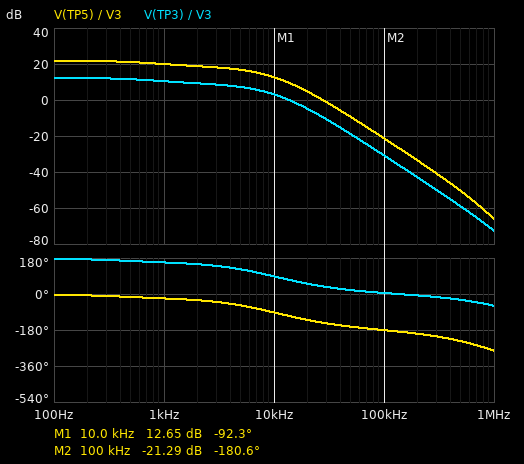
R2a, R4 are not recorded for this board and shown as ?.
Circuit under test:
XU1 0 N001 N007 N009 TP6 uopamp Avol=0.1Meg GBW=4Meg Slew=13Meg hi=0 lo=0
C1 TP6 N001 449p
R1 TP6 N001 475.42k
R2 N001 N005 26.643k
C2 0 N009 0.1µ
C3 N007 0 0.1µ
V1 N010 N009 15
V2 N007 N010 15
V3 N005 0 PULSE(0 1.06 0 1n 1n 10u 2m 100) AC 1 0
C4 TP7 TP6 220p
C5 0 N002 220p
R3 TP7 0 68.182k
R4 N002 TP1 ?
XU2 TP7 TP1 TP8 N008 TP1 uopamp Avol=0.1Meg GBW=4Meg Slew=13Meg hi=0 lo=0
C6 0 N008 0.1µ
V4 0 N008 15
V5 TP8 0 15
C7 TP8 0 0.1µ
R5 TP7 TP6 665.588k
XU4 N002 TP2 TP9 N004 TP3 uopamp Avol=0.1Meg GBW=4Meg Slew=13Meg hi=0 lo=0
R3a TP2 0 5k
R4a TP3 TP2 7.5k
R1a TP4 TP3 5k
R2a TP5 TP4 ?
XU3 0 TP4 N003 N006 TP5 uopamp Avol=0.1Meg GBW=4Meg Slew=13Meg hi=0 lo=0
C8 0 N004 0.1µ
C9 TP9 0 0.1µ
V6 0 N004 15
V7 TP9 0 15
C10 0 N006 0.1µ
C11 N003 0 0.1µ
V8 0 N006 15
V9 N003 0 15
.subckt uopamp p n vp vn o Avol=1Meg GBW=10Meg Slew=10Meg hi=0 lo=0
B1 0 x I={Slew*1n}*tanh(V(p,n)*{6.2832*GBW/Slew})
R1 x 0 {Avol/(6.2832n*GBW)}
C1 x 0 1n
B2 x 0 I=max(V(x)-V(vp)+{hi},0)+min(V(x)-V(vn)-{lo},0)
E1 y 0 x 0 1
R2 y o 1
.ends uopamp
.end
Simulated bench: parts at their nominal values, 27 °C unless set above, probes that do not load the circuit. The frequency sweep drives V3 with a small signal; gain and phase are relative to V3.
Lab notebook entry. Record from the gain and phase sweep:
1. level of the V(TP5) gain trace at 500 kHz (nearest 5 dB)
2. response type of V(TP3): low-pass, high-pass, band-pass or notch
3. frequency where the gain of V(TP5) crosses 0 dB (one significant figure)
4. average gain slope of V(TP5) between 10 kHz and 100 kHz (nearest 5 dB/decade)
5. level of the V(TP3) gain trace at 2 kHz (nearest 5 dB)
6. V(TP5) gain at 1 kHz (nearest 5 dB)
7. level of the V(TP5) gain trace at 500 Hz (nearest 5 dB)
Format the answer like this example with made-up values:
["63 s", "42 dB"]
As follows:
["-50 dB", "low-pass", "30 kHz", "-35 dB/decade", "10 dB", "20 dB", "20 dB"]
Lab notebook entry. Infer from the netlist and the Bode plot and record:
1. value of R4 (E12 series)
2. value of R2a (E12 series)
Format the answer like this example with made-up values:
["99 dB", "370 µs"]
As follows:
["82 kΩ", "15 kΩ"]
